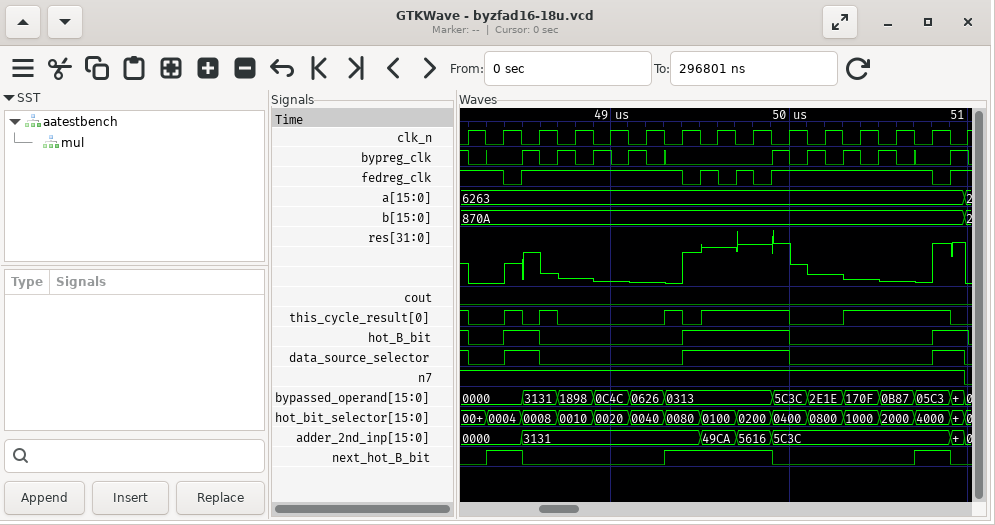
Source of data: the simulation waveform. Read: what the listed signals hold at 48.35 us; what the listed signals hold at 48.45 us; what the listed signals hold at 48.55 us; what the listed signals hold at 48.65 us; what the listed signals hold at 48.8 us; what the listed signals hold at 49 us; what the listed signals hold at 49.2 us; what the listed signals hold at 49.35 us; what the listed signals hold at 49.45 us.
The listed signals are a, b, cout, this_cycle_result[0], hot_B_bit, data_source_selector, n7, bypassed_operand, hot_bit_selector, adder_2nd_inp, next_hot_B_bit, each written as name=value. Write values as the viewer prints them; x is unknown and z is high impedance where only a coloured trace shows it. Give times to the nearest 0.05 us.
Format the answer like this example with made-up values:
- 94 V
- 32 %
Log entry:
- a=6263, b=870A, cout=0, this_cycle_result[0]=0, hot_B_bit=0, data_source_selector=0, n7=1, bypassed_operand=0000, hot_bit_selector=0004, adder_2nd_inp=0000, next_hot_B_bit=1
- a=6263, b=870A, cout=0, this_cycle_result[0]=1, hot_B_bit=1, data_source_selector=1, n7=1, bypassed_operand=0000, hot_bit_selector=0004, adder_2nd_inp=0000, next_hot_B_bit=1
- a=6263, b=870A, cout=0, this_cycle_result[0]=0, hot_B_bit=1, data_source_selector=1, n7=1, bypassed_operand=3131, hot_bit_selector=0008, adder_2nd_inp=3131, next_hot_B_bit=0
- a=6263, b=870A, cout=0, this_cycle_result[0]=1, hot_B_bit=0, data_source_selector=0, n7=1, bypassed_operand=3131, hot_bit_selector=0008, adder_2nd_inp=3131, next_hot_B_bit=0
- a=6263, b=870A, cout=0, this_cycle_result[0]=0, hot_B_bit=0, data_source_selector=0, n7=1, bypassed_operand=1898, hot_bit_selector=0010, adder_2nd_inp=3131, next_hot_B_bit=0
- a=6263, b=870A, cout=0, this_cycle_result[0]=0, hot_B_bit=0, data_source_selector=0, n7=1, bypassed_operand=0C4C, hot_bit_selector=0020, adder_2nd_inp=3131, next_hot_B_bit=0
- a=6263, b=870A, cout=0, this_cycle_result[0]=0, hot_B_bit=0, data_source_selector=0, n7=1, bypassed_operand=0626, hot_bit_selector=0040, adder_2nd_inp=3131, next_hot_B_bit=0
- a=6263, b=870A, cout=0, this_cycle_result[0]=1, hot_B_bit=0, data_source_selector=0, n7=1, bypassed_operand=0313, hot_bit_selector=0080, adder_2nd_inp=3131, next_hot_B_bit=1
- a=6263, b=870A, cout=0, this_cycle_result[0]=0, hot_B_bit=1, data_source_selector=1, n7=1, bypassed_operand=0313, hot_bit_selector=0080, adder_2nd_inp=3131, next_hot_B_bit=1
